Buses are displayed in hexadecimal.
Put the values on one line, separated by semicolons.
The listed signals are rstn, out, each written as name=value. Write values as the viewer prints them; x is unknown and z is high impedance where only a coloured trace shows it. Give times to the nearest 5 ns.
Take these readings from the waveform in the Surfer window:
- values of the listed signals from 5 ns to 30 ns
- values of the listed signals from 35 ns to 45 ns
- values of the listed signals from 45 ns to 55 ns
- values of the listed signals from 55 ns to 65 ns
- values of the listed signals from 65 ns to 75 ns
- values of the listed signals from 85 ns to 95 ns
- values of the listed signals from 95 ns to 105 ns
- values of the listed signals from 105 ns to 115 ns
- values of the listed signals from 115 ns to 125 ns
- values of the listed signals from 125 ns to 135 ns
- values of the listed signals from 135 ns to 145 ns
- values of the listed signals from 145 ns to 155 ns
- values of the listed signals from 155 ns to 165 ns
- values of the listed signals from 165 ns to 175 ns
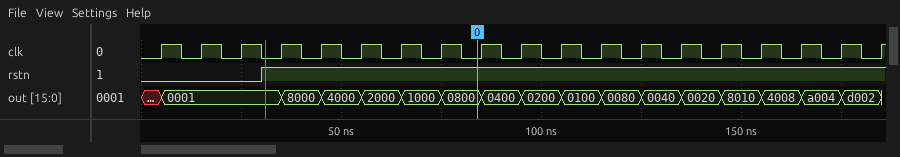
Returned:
rstn=0, out=0001; rstn=1, out=8000; rstn=1, out=4000; rstn=1, out=2000; rstn=1, out=1000; rstn=1, out=0400; rstn=1, out=0200; rstn=1, out=0100; rstn=1, out=0080; rstn=1, out=0040; rstn=1, out=0020; rstn=1, out=8010; rstn=1, out=4008; rstn=1, out=a004
